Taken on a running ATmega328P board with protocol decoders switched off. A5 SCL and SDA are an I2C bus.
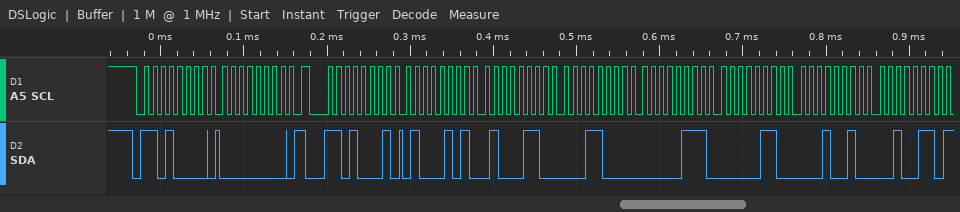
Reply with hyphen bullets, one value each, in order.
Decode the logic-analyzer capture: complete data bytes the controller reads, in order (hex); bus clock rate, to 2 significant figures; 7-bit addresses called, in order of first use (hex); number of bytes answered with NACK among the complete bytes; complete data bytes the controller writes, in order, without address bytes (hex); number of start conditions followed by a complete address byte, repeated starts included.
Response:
- 45 46 18 07 06 12 26
- 100 kHz
- 0x68
- 1
- 00
- 2
